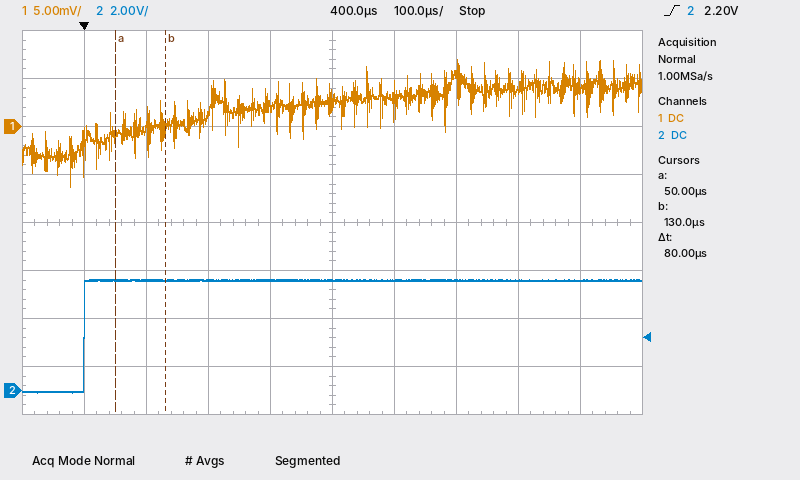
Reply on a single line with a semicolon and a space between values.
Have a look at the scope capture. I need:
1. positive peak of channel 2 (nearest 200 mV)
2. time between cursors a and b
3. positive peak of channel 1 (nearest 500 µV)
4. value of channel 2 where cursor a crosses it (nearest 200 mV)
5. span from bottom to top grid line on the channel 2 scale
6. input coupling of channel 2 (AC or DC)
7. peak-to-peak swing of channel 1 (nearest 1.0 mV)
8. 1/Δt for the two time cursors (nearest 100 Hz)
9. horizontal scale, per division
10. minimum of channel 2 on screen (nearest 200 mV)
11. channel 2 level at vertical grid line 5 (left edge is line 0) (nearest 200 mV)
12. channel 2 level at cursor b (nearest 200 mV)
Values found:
4.6 V; 80 µs; 7.0 mV; 4.6 V; 16 V; DC; 13.0 mV; 12.5 kHz; 100 µs; 0.0 V; 4.6 V; 4.6 V
